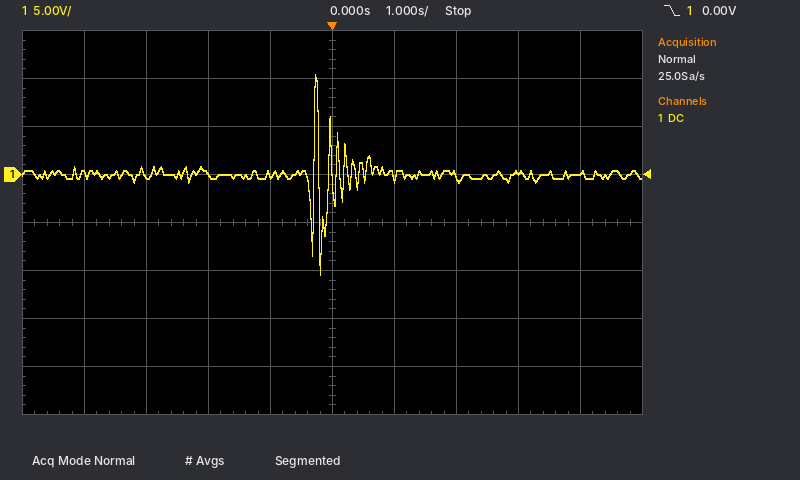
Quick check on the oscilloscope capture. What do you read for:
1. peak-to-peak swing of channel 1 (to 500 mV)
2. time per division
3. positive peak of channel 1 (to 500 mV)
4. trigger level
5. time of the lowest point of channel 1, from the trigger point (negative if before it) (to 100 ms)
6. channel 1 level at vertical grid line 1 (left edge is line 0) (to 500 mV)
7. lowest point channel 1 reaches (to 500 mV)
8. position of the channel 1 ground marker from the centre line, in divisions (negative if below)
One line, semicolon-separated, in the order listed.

21.0 V; 1 s; 10.5 V; 0.00 V; -200 ms; 0.0 V; -10.5 V; +1.0 div
